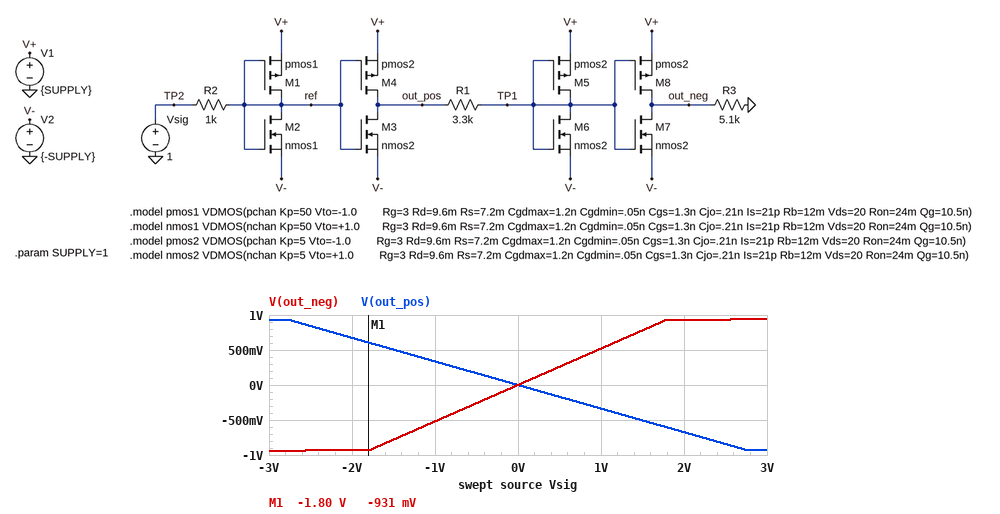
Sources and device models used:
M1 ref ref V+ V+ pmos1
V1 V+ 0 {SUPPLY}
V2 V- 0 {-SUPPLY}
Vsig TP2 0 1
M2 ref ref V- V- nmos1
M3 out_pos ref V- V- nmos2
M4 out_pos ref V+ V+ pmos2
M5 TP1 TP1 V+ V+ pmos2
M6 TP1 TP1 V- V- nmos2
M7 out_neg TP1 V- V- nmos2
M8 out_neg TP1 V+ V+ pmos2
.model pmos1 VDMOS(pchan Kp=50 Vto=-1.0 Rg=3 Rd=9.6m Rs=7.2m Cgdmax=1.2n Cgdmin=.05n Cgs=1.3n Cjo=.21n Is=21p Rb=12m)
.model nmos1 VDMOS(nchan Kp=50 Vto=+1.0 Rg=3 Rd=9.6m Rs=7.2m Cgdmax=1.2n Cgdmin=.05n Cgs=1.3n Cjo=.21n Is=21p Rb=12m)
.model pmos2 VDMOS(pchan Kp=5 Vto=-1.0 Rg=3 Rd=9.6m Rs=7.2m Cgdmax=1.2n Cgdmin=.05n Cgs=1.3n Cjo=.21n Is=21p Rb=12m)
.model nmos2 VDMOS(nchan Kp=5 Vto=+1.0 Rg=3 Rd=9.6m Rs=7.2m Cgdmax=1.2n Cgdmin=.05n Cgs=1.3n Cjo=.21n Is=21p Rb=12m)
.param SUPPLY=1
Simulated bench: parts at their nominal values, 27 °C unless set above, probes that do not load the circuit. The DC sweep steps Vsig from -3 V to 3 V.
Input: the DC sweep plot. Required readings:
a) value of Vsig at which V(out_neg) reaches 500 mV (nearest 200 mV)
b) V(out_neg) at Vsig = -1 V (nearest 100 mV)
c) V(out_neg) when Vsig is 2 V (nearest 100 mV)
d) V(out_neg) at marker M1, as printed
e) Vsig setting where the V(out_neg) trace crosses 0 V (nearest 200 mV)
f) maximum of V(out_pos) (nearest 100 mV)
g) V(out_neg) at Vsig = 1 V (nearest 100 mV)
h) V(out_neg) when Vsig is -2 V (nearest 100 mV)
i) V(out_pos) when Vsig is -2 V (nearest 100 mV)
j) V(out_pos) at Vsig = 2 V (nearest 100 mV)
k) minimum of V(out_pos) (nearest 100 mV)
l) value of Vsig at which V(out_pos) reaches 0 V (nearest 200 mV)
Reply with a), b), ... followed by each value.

a) 1.0 V
b) -500 mV
c) 900 mV
d) -931 mV
e) 0 V
f) 900 mV
g) 500 mV
h) -900 mV
i) 700 mV
j) -700 mV
k) -900 mV
l) 0 V
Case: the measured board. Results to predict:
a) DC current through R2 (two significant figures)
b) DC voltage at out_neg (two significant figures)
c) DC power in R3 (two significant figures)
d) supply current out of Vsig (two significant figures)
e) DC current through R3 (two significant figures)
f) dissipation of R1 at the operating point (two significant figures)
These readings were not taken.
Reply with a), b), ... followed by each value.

a) 1.0 mA
b) 520 mV
c) 53 µW
d) 1.0 mA
e) 100 µA
f) 34 µW
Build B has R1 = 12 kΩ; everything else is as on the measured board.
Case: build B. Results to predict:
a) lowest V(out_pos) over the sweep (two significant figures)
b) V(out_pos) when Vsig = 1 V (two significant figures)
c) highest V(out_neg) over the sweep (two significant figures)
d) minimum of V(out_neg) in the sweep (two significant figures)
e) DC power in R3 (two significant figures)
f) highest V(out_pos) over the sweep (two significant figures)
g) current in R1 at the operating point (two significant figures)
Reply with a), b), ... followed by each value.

a) -940 mV
b) -930 mV
c) 400 mV
d) -400 mV
e) 31 µW
f) 940 mV
g) 78 µA
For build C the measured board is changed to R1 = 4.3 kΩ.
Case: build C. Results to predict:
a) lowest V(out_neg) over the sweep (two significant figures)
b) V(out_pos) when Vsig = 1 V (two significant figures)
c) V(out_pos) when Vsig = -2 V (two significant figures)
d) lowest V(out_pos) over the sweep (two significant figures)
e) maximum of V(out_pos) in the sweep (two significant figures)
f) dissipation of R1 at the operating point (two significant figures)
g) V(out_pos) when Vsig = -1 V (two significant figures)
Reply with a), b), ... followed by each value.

a) -930 mV
b) -440 mV
c) 880 mV
d) -940 mV
e) 940 mV
f) 45 µW
g) 440 mV
